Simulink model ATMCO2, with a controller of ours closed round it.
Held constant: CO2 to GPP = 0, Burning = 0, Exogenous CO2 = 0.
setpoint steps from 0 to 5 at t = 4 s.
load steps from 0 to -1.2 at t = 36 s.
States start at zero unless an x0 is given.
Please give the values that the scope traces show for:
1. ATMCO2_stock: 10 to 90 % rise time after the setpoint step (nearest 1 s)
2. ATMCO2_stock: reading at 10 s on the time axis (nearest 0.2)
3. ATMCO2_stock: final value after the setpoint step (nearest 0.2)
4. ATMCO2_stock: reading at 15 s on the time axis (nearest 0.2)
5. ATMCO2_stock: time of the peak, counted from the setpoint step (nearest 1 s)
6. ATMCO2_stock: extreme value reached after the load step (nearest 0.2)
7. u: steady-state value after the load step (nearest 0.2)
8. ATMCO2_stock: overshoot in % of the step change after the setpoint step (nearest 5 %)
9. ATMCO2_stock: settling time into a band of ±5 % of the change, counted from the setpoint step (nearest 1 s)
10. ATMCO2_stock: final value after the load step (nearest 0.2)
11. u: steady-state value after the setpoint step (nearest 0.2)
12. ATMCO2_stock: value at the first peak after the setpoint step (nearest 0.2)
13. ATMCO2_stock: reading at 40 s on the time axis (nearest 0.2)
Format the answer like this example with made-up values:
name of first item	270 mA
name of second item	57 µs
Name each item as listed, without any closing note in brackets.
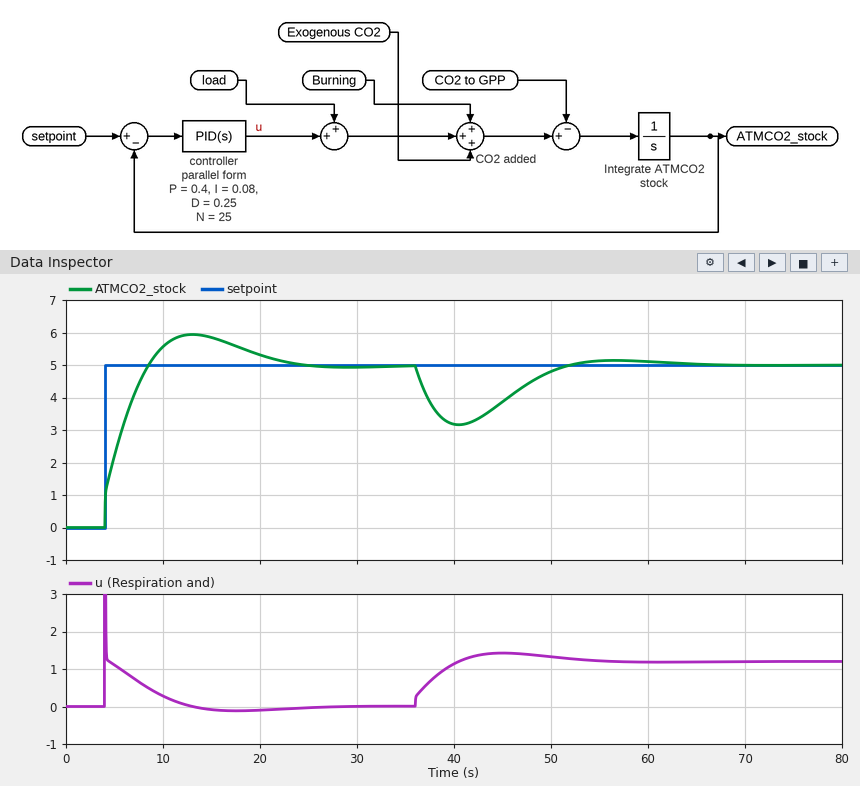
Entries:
ATMCO2_stock: 10 to 90 % rise time after the setpoint step	4 s
ATMCO2_stock: reading at 10 s on the time axis	5.6
ATMCO2_stock: final value after the setpoint step	5.0
ATMCO2_stock: reading at 15 s on the time axis	5.8
ATMCO2_stock: time of the peak, counted from the setpoint step	9 s
ATMCO2_stock: extreme value reached after the load step	3.2
u: steady-state value after the load step	1.2
ATMCO2_stock: overshoot in % of the step change after the setpoint step	20 %
ATMCO2_stock: settling time into a band of ±5 % of the change, counted from the setpoint step	17 s
ATMCO2_stock: final value after the load step	5.0
u: steady-state value after the setpoint step	0.0
ATMCO2_stock: value at the first peak after the setpoint step	6.0
ATMCO2_stock: reading at 40 s on the time axis	3.2
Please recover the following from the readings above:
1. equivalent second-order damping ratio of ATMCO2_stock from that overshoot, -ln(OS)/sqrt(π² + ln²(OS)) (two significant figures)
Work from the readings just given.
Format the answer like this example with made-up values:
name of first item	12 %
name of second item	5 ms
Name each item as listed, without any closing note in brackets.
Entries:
equivalent second-order damping ratio of ATMCO2_stock from that overshoot, -ln(OS)/sqrt(π² + ln²(OS))	0.46
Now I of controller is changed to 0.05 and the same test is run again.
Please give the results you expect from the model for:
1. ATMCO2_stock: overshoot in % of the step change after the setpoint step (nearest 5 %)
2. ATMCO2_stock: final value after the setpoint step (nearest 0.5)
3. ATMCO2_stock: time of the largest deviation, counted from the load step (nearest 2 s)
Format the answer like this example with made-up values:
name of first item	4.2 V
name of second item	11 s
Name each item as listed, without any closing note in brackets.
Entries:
ATMCO2_stock: overshoot in % of the step change after the setpoint step	15 %
ATMCO2_stock: final value after the setpoint step	5.0
ATMCO2_stock: time of the largest deviation, counted from the load step	6 s
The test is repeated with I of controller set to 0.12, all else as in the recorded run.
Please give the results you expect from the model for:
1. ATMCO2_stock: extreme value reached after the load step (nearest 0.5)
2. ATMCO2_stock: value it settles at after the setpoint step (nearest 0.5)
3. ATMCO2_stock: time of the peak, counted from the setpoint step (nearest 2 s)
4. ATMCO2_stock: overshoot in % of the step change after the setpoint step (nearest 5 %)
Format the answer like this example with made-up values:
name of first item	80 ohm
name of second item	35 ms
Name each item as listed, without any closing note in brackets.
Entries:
ATMCO2_stock: extreme value reached after the load step	3.5
ATMCO2_stock: value it settles at after the setpoint step	5.0
ATMCO2_stock: time of the peak, counted from the setpoint step	8 s
ATMCO2_stock: overshoot in % of the step change after the setpoint step	25 %
